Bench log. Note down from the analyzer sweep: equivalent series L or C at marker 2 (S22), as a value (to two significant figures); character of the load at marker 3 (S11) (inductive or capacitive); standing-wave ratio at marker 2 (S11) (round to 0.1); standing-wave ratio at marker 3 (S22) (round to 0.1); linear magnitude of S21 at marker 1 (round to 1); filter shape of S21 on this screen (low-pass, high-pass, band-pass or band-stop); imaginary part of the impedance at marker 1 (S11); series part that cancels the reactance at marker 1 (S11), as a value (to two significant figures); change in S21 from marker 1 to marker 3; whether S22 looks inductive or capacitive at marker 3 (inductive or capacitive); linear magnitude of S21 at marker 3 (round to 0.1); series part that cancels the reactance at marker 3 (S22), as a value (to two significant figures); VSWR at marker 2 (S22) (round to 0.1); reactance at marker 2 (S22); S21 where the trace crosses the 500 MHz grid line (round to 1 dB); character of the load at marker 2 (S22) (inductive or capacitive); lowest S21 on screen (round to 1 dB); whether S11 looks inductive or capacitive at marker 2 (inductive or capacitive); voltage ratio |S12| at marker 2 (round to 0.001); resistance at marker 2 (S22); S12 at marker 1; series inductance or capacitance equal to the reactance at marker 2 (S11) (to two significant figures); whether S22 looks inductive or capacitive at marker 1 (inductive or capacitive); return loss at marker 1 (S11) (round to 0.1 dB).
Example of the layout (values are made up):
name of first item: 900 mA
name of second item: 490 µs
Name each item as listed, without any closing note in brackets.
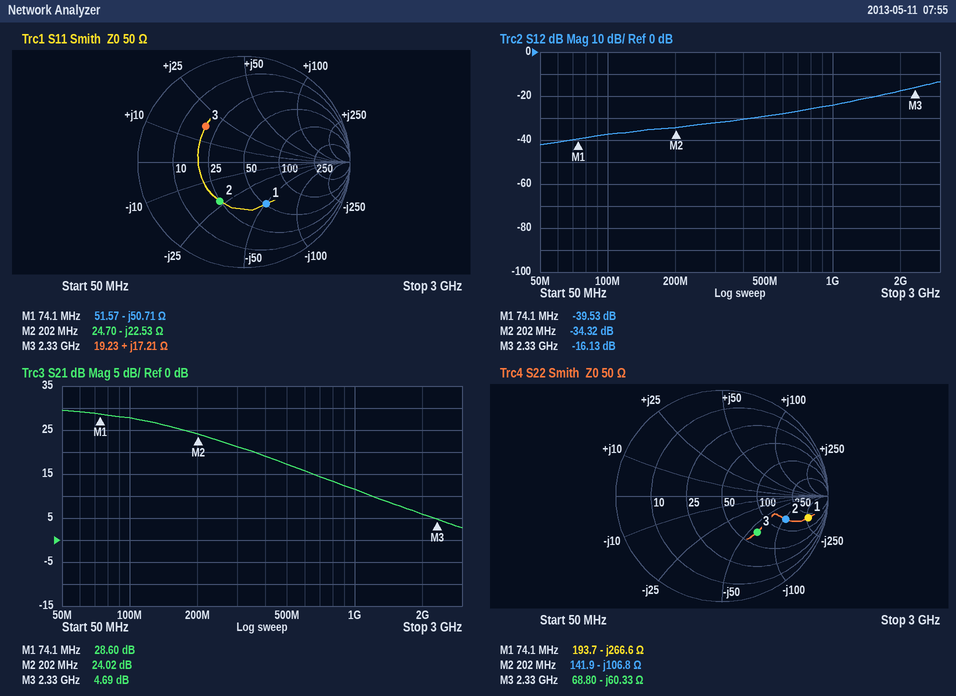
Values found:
equivalent series L or C at marker 2 (S22), as a value: 7.4 pF
character of the load at marker 3 (S11): inductive
standing-wave ratio at marker 2 (S11): 2.5
standing-wave ratio at marker 3 (S22): 2.8
linear magnitude of S21 at marker 1: 27
filter shape of S21 on this screen: low-pass
imaginary part of the impedance at marker 1: -50.71 Ω
series part that cancels the reactance at marker 1 (S11), as a value: 110 nH
change in S21 from marker 1 to marker 3: -23.91 dB
whether S22 looks inductive or capacitive at marker 3: capacitive
linear magnitude of S21 at marker 3: 1.7
series part that cancels the reactance at marker 3 (S22), as a value: 4.1 nH
VSWR at marker 2 (S22): 4.6
reactance at marker 2: -106.8 Ω
S21 where the trace crosses the 500 MHz grid line: 17 dB
character of the load at marker 2 (S22): capacitive
lowest S21 on screen: 3 dB
whether S11 looks inductive or capacitive at marker 2: capacitive
voltage ratio |S12| at marker 2: 0.019
resistance at marker 2: 141.9 Ω
S12 at marker 1: -39.53 dB
series inductance or capacitance equal to the reactance at marker 2 (S11): 35 pF
whether S22 looks inductive or capacitive at marker 1: capacitive
return loss at marker 1 (S11): 7.0 dB
